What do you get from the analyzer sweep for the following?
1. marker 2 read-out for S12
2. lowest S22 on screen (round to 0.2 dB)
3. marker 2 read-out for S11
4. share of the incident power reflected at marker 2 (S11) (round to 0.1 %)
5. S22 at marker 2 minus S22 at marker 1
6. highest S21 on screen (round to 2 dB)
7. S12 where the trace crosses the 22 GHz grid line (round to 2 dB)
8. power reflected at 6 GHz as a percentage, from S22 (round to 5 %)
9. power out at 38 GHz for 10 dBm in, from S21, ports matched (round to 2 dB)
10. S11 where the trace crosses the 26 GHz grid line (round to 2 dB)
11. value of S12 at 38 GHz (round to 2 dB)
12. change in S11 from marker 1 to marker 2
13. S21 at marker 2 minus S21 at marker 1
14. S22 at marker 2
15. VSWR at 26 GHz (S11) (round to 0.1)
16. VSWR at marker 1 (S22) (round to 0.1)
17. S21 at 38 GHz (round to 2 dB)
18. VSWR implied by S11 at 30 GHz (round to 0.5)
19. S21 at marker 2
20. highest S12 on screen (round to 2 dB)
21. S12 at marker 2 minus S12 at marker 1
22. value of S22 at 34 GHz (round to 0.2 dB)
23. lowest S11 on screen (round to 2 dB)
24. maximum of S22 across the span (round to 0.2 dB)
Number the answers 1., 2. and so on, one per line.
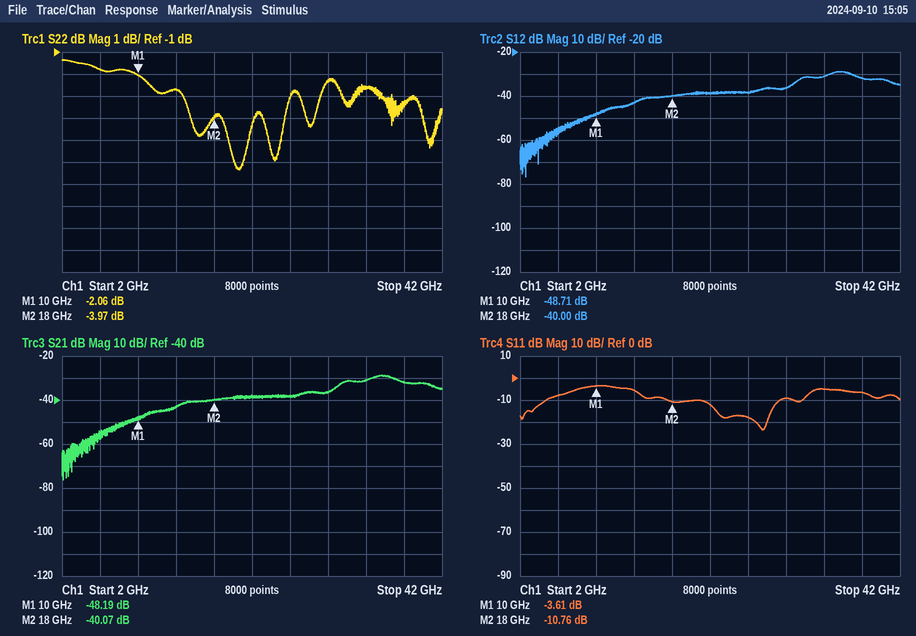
1. -40.00 dB
2. -6.4 dB
3. -10.76 dB
4. 8.4 %
5. -1.91 dB
6. -28 dB
7. -38 dB
8. 65 %
9. -22 dBm
10. -18 dB
11. -32 dB
12. -7.15 dB
13. 8.12 dB
14. -3.97 dB
15. 1.3
16. 8.5
17. -32 dB
18. 2.0
19. -40.07 dB
20. -28 dB
21. 8.71 dB
22. -2.6 dB
23. -24 dB
24. -1.4 dB
